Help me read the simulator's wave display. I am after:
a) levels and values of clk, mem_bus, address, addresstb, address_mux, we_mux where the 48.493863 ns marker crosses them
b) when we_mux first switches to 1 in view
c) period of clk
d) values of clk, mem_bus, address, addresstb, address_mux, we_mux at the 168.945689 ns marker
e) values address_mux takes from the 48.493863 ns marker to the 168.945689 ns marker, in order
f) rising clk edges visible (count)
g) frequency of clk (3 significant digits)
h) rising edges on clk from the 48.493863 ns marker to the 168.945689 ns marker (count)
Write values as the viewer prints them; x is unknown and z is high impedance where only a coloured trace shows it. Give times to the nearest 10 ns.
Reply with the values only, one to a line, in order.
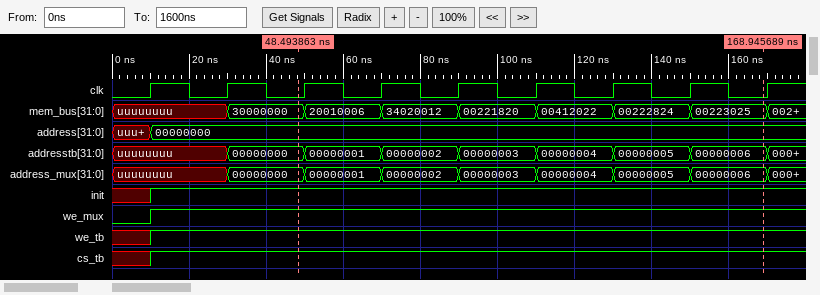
clk=0, mem_bus=30000000, address=00000000, addresstb=00000000, address_mux=00000000, we_mux=1
10 ns
20 ns
clk=0, mem_bus=00223025, address=00000000, addresstb=00000006, address_mux=00000006, we_mux=1
00000000, 00000001, 00000002, 00000003, 00000004, 00000005, 00000006
9
50.0 MHz
6
